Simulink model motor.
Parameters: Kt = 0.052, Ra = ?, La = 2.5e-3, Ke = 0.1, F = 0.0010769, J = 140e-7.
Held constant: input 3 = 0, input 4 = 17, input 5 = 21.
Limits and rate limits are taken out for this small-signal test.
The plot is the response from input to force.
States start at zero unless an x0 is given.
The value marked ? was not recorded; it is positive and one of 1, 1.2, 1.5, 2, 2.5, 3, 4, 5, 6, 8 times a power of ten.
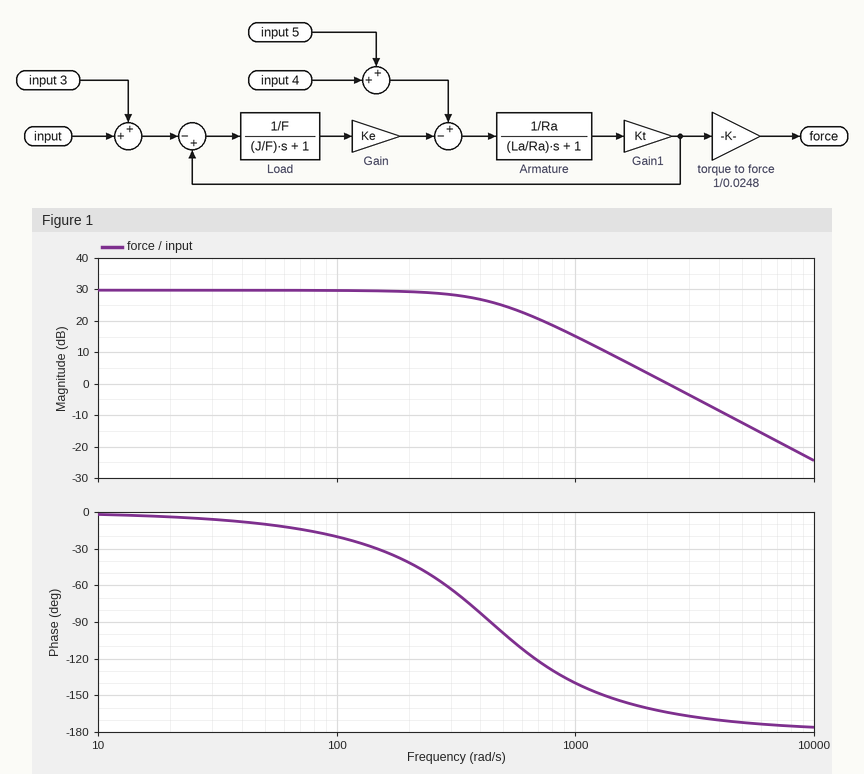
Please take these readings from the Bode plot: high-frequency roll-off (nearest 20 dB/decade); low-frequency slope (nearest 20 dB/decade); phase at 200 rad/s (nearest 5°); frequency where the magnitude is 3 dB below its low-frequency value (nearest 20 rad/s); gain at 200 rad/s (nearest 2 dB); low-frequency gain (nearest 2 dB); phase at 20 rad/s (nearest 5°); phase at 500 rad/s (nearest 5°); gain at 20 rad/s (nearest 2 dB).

-40 dB/decade
0 dB/decade
-40°
400 rad/s
30 dB
30 dB
-5°
-100°
30 dB
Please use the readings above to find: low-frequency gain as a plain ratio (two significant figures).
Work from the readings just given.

32
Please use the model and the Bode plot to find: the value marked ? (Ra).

1.5
